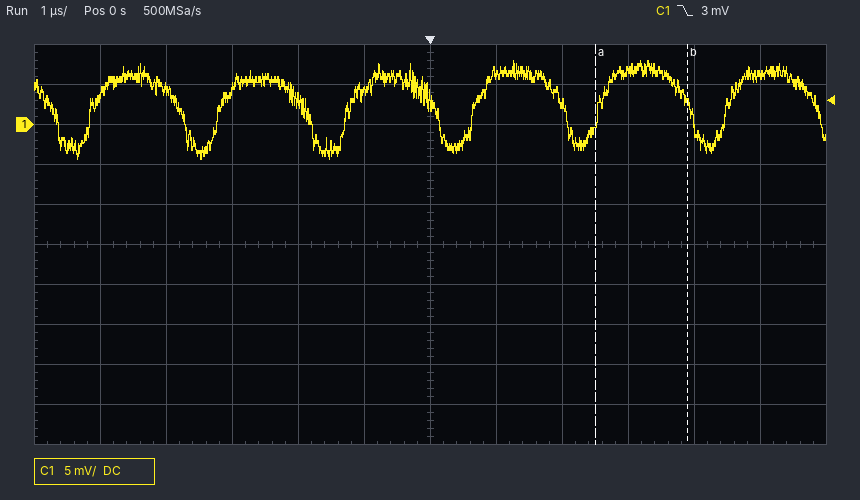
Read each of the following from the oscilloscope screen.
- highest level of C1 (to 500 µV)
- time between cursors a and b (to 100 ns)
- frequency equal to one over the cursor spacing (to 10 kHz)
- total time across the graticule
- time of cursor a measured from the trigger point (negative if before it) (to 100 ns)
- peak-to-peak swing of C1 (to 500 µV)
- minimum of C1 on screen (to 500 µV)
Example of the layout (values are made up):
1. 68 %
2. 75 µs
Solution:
1. 8.0 mV
2. 1.4 µs
3. 710 kHz
4. 12 µs
5. +2.5 µs
6. 12.5 mV
7. -4.5 mV
